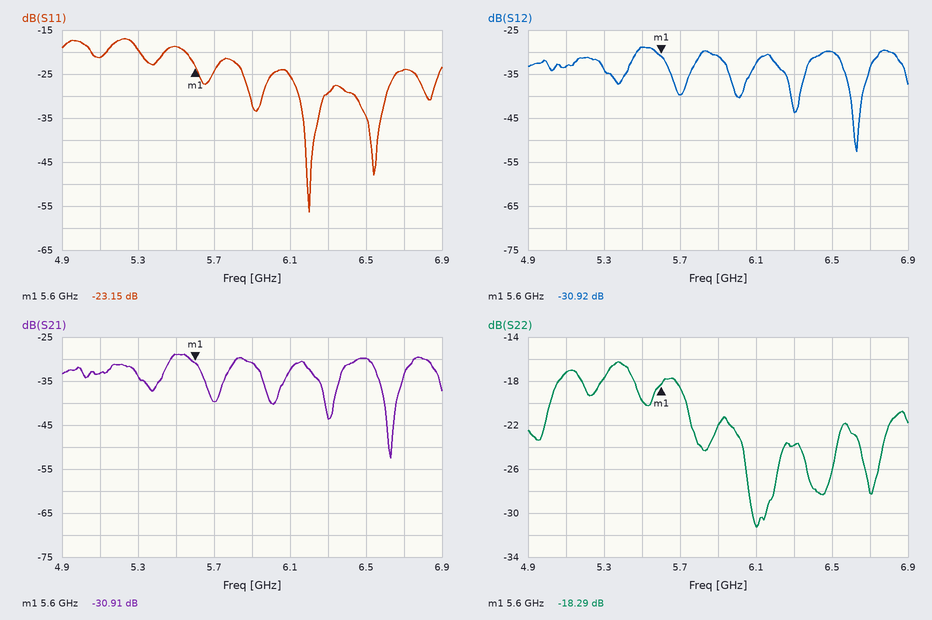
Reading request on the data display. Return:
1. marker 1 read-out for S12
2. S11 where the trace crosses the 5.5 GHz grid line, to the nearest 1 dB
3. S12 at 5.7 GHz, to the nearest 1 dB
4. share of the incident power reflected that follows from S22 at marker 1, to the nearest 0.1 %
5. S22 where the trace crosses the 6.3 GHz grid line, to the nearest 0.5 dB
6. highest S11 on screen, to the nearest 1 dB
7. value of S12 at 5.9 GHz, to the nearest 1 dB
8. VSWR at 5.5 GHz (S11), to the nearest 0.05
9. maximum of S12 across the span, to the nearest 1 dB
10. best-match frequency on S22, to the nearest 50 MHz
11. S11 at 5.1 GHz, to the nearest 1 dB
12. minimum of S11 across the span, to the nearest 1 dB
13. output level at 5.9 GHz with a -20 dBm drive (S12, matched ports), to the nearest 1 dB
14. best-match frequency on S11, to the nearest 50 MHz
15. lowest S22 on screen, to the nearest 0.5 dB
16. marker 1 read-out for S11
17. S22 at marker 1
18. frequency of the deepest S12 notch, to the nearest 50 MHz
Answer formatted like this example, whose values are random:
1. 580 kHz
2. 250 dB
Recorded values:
1. -30.92 dB
2. -19 dB
3. -40 dB
4. 1.5 %
5. -24.0 dB
6. -17 dB
7. -31 dB
8. 1.25
9. -29 dB
10. 6.10 GHz
11. -21 dB
12. -56 dB
13. -51 dBm
14. 6.20 GHz
15. -31.5 dB
16. -23.15 dB
17. -18.29 dB
18. 6.65 GHz
